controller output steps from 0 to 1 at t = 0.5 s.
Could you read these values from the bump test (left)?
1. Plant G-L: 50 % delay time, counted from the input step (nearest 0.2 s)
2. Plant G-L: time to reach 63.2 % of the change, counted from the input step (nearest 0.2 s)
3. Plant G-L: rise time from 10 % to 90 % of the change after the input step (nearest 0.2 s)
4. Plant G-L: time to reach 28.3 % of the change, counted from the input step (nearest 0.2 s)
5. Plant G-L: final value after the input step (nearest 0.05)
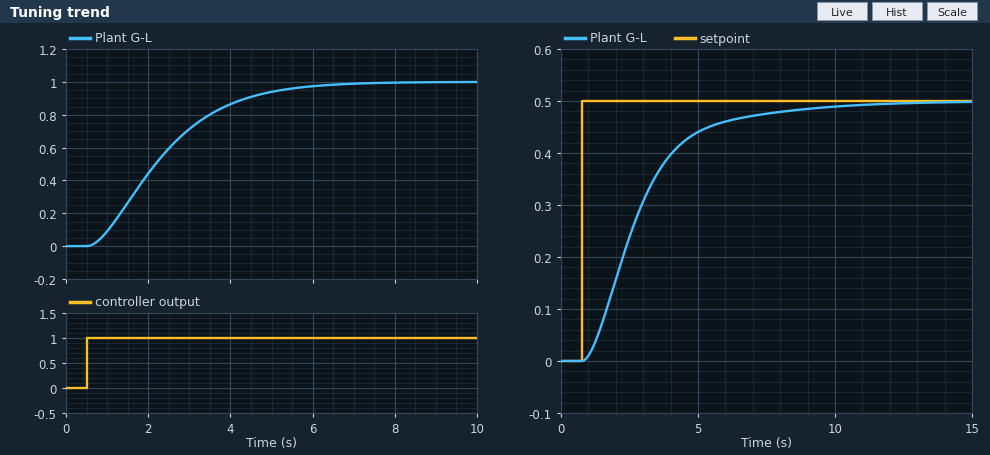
1.6 s
2.2 s
3.4 s
1.0 s
1.00
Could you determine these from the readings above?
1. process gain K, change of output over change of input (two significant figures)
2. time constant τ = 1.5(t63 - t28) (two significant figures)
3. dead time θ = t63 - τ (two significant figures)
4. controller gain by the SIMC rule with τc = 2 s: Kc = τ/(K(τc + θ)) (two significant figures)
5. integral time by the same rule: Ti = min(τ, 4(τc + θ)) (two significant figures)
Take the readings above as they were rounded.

1.0
1.8 s
0.40 s
0.75
1.8 s
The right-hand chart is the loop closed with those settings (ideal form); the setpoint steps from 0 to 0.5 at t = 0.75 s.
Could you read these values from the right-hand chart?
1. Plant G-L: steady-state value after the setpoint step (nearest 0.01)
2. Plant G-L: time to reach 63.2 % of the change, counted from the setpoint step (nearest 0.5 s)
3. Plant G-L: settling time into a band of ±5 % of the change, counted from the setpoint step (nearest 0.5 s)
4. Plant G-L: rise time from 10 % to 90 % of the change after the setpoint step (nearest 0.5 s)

0.50
2.5 s
6.5 s
4.0 s
